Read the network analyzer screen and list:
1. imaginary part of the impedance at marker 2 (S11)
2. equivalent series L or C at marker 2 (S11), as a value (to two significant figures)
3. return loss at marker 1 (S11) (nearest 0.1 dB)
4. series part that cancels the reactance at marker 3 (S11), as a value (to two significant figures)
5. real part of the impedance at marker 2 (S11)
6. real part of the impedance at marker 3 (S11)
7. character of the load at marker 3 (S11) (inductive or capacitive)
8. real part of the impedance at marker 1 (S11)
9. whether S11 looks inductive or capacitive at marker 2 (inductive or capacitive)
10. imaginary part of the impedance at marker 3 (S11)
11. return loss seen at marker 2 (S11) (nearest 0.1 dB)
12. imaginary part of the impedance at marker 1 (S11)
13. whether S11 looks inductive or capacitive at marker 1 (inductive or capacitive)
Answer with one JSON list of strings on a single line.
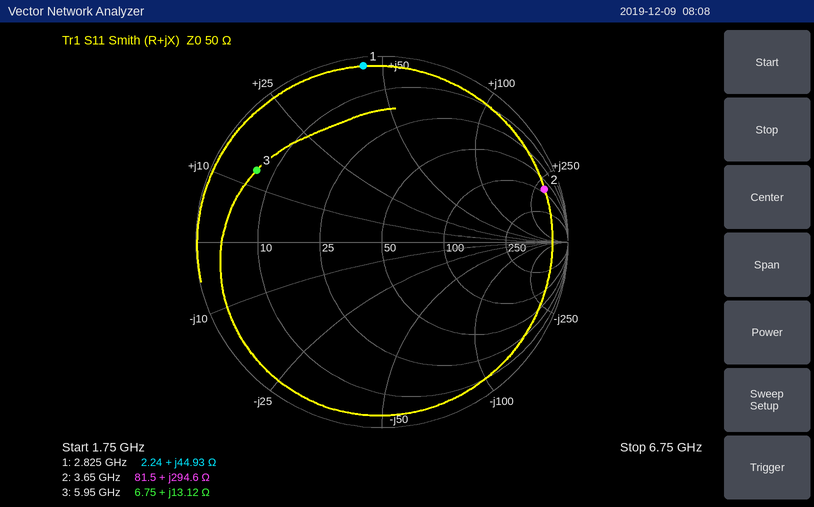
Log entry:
["+294.6 Ω", "13 nH", "0.4 dB", "2.0 pF", "81.5 Ω", "6.75 Ω", "inductive", "2.24 Ω", "inductive", "+13.12 Ω", "0.7 dB", "+44.93 Ω", "inductive"]
